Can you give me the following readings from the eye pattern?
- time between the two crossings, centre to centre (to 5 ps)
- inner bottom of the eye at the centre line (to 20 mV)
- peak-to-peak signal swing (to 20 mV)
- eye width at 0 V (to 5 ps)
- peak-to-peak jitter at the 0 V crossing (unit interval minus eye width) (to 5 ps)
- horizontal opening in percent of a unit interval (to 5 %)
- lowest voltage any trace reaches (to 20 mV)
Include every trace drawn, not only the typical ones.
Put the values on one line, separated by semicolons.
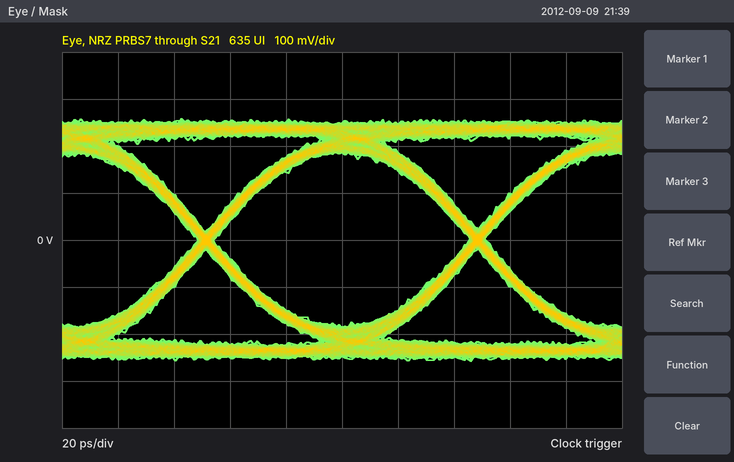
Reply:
95 ps; -180 mV; 520 mV; 90 ps; 5 ps; 95 %; -260 mV
